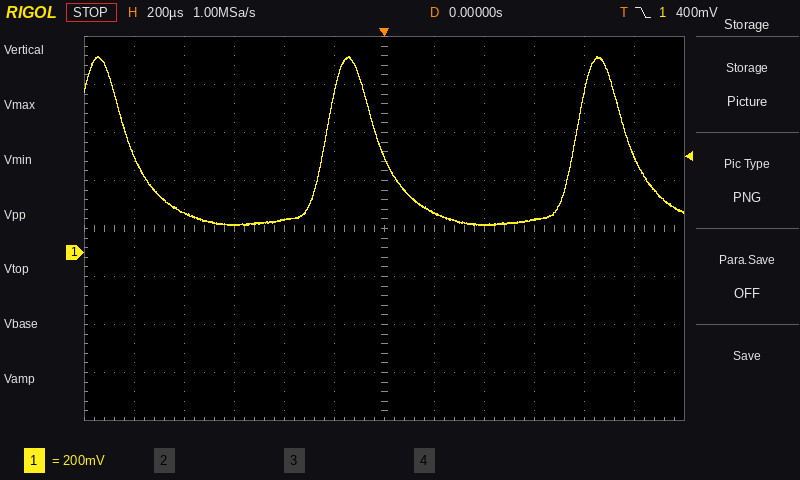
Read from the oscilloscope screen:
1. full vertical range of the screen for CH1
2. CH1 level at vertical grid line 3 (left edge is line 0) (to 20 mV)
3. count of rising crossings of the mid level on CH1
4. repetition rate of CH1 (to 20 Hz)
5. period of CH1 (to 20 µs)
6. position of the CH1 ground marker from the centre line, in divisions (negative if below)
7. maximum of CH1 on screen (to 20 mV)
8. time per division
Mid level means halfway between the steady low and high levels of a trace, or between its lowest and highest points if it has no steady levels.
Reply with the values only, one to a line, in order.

1.6 V
120 mV
2
1.00 kHz
1.00 ms
-0.5 div
820 mV
200 µs
